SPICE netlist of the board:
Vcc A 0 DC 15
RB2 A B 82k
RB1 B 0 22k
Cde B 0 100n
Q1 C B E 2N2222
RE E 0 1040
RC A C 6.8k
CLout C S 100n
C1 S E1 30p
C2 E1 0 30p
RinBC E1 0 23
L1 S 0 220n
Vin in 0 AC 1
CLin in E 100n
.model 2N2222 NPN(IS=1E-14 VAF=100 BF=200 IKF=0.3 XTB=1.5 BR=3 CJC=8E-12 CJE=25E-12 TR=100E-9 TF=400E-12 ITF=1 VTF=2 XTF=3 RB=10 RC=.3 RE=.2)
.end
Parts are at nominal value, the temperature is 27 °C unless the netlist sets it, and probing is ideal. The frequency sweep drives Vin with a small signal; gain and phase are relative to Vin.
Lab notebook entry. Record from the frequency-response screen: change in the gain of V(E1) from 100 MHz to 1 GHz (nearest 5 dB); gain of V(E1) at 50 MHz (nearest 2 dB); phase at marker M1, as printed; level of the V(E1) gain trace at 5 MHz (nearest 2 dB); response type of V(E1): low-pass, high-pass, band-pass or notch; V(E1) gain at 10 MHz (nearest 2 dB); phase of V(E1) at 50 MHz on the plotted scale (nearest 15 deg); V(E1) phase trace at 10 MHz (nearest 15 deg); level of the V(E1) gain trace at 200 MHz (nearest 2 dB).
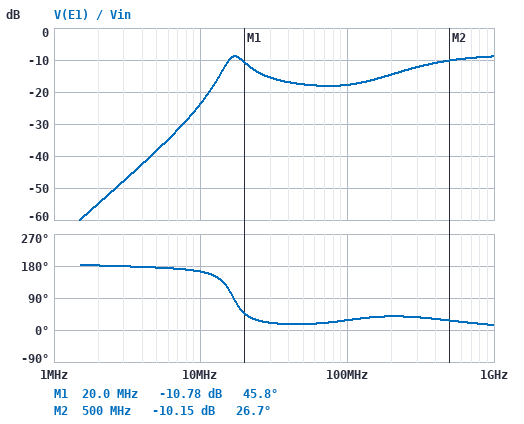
10 dB
-18 dB
45.8 deg
-38 dB
high-pass
-24 dB
15 deg
165 deg
-14 dB
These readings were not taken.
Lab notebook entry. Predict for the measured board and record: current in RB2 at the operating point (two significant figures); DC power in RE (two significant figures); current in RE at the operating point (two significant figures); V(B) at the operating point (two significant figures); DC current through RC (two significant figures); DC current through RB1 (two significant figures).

150 µA
3.9 mW
1.9 mA
2.7 V
1.9 mA
120 µA
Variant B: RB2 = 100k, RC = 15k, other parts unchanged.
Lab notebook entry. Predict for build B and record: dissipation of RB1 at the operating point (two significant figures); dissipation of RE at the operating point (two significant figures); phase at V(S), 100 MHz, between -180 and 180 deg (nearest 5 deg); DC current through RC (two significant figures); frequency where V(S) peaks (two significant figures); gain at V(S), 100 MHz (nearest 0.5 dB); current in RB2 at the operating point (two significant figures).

130 µW
1.0 mW
15 deg
930 µA
12 MHz
-10.0 dB
130 µA
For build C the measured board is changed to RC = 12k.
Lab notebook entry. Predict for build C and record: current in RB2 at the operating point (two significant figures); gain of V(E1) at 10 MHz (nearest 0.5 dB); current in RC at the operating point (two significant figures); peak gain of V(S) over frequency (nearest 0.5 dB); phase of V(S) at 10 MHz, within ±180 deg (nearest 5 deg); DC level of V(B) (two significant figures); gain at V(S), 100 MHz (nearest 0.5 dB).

160 µA
-25.5 dB
1.1 mA
2.0 dB
25 deg
1.9 V
-9.0 dB
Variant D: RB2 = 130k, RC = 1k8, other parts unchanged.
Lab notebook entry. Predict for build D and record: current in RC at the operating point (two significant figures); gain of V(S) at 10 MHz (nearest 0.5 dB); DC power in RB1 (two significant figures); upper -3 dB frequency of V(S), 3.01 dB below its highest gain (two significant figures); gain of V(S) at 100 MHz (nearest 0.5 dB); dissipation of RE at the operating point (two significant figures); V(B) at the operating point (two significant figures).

1.3 mA
-3.0 dB
190 µW
67 MHz
12.0 dB
1.9 mW
2.1 V
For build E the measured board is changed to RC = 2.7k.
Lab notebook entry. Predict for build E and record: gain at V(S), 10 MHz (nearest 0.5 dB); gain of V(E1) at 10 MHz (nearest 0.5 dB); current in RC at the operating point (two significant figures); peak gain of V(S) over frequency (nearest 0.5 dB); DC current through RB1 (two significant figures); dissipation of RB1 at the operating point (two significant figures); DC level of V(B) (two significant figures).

1.5 dB
-26.0 dB
2.2 mA
29.0 dB
140 µA
410 µW
3.0 V
